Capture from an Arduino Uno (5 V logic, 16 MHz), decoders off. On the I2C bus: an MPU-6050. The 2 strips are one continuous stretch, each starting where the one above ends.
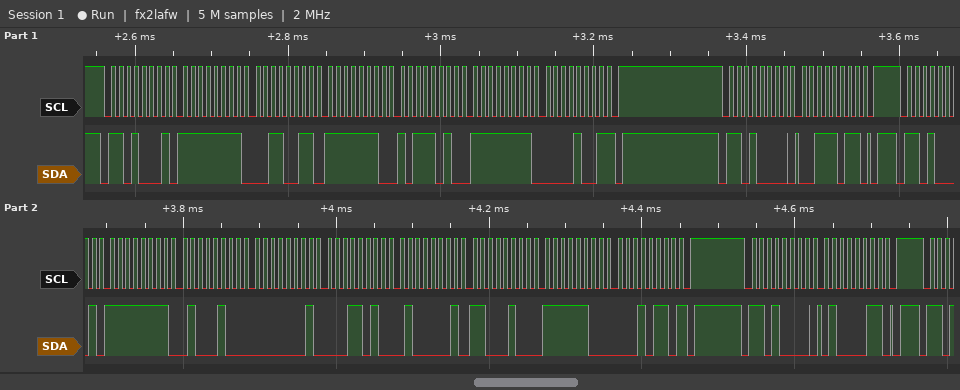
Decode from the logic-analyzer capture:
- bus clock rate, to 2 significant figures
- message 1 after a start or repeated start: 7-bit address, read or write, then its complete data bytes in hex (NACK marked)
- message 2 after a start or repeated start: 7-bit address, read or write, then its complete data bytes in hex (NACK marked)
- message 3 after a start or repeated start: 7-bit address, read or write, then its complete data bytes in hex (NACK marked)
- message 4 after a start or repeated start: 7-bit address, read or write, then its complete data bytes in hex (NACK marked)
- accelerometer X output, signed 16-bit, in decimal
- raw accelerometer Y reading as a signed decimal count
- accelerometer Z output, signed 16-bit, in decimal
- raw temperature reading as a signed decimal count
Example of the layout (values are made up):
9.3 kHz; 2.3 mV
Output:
100 kHz; 0x68 read: FF 33 FE BA FF 09 NACK; 0x68 write: 3B; 0x68 read: FF 44 01 1A 41 C4 FC 16 NACK; 0x68 write: 43; -188; 282; 16836; -1002
